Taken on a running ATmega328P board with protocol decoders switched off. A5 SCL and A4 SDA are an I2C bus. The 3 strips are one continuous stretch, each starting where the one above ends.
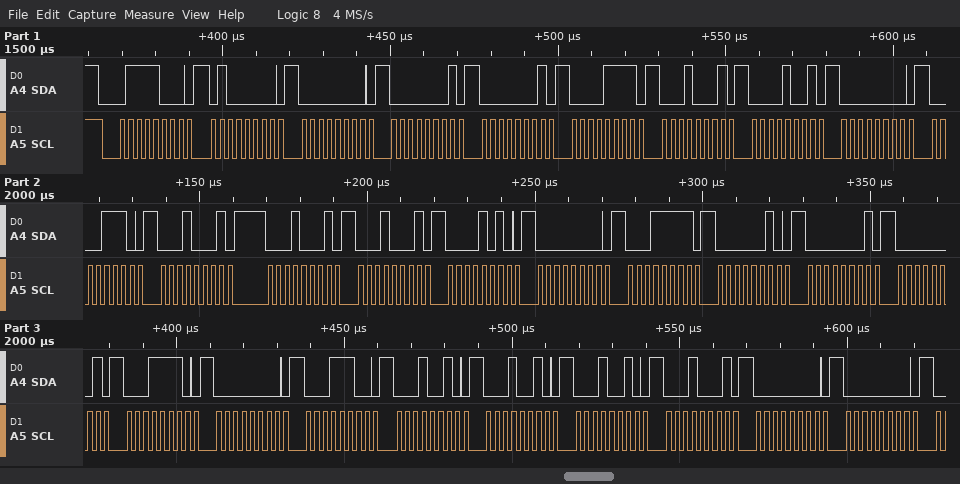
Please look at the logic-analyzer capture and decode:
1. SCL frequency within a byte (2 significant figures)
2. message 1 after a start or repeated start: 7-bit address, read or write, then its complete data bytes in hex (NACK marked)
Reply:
400 kHz
0x3C write: 40 00 01 01 0F 11 09 00 0E 11 11 11 0A 00 1F 02 01 01 1E 00 1C 12 12 12 11 00 00
